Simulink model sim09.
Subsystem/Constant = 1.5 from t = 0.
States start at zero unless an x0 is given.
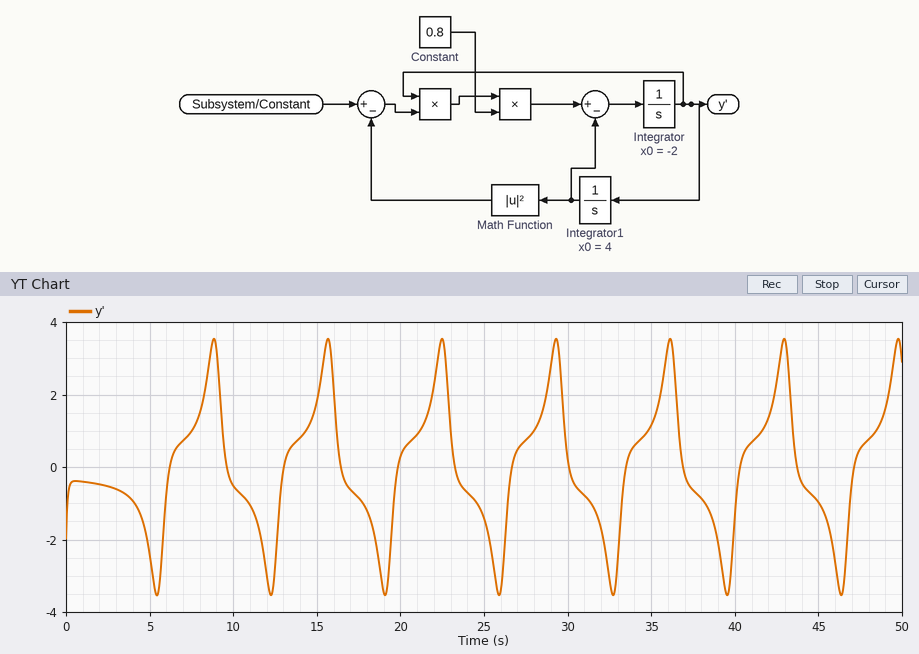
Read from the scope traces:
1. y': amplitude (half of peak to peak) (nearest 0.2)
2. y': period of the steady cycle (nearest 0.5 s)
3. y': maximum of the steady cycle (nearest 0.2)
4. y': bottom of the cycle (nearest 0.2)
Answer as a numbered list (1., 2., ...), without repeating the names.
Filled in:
1. 3.6
2. 7.0 s
3. 3.6
4. -3.6
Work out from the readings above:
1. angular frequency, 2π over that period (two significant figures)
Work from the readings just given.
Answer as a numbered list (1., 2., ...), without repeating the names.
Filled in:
1. 0.90 rad/s
